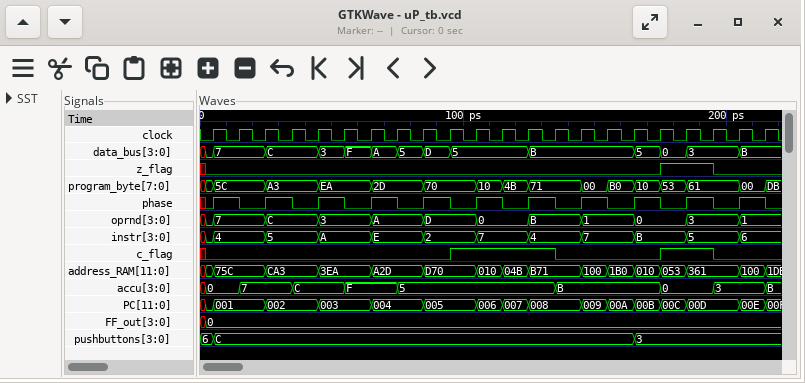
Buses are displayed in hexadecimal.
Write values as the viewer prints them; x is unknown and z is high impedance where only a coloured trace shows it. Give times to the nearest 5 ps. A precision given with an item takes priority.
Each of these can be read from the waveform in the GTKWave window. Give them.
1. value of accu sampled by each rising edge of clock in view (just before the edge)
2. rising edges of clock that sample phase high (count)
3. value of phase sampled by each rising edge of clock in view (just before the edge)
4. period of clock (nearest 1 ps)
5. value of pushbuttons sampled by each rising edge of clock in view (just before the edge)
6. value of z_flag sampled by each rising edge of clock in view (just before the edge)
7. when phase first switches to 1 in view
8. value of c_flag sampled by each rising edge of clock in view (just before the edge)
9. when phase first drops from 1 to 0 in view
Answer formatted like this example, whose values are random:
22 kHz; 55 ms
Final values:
0, 0, 7, 7, C, C, F, F, 5, 5, 5, 5, 5, 5, B, B, B, B, 0, 0, 3, 3; 11; 0 1 0 1 0 1 0 1 0 1 0 1 0 1 0 1 0 1 0 1 0 1; 10 ps; 6, C, C, C, C, C, C, C, C, C, C, C, C, C, C, C, C, 3, 3, 3, 3, 3; 0 0 0 0 0 0 0 0 0 0 0 0 0 0 0 0 0 0 1 1 0 0; 5 ps; 0 0 0 0 0 0 0 0 0 0 1 1 1 1 0 0 0 0 1 1 0 0; 15 ps
